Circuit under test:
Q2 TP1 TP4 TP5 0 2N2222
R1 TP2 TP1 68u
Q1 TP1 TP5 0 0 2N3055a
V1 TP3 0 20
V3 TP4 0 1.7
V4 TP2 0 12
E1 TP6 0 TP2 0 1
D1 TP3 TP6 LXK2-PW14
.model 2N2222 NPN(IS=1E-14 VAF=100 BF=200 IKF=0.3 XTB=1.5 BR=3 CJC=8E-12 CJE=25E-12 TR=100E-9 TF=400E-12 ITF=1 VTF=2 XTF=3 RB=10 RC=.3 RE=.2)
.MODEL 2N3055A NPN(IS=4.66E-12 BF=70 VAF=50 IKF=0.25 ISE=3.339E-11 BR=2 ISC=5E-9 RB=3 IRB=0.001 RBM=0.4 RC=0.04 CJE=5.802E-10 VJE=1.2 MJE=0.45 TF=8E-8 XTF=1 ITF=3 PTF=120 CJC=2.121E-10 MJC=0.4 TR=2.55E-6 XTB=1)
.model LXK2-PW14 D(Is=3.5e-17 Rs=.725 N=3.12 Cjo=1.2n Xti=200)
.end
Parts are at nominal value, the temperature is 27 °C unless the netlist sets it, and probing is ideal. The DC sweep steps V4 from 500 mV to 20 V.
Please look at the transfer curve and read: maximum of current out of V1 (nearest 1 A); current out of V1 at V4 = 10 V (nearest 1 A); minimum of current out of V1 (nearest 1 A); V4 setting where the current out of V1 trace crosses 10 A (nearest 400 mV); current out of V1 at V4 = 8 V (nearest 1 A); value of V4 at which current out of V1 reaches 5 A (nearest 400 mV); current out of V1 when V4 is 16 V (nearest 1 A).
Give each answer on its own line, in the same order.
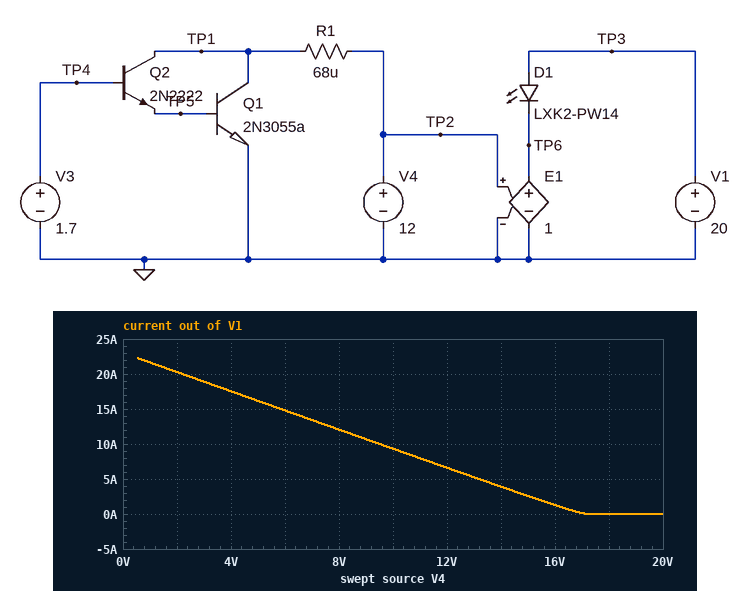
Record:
22 A
9 A
0 A
9.6 V
12 A
13.2 V
1 A
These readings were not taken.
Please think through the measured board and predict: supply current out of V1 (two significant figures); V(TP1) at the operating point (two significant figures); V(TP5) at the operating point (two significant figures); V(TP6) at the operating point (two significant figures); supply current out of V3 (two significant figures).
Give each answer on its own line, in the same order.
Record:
6.6 A
12 V
850 mV
12 V
1.4 mA
